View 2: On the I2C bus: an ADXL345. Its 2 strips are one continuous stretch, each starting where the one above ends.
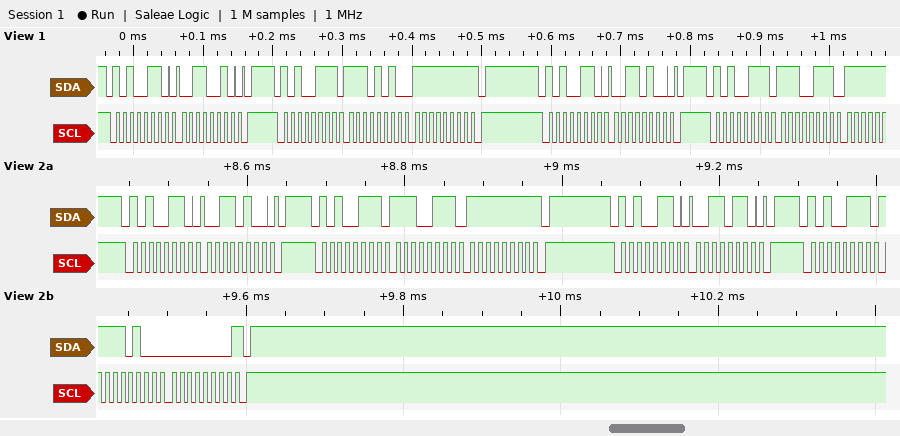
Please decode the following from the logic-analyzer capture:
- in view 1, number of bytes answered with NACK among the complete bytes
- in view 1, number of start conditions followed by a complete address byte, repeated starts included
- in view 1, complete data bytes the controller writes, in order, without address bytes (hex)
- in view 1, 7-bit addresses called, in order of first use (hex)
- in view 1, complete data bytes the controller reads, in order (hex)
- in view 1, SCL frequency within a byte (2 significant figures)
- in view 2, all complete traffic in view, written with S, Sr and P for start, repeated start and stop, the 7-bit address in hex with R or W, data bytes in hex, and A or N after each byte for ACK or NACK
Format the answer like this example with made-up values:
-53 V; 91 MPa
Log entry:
1; 4; 32 34; 0x53; EA FF E7; 100 kHz; S 53W A 34 A P S 53R A E7 A FF N P S 53W A 36 A P S 53R A F4 A 00 N P
